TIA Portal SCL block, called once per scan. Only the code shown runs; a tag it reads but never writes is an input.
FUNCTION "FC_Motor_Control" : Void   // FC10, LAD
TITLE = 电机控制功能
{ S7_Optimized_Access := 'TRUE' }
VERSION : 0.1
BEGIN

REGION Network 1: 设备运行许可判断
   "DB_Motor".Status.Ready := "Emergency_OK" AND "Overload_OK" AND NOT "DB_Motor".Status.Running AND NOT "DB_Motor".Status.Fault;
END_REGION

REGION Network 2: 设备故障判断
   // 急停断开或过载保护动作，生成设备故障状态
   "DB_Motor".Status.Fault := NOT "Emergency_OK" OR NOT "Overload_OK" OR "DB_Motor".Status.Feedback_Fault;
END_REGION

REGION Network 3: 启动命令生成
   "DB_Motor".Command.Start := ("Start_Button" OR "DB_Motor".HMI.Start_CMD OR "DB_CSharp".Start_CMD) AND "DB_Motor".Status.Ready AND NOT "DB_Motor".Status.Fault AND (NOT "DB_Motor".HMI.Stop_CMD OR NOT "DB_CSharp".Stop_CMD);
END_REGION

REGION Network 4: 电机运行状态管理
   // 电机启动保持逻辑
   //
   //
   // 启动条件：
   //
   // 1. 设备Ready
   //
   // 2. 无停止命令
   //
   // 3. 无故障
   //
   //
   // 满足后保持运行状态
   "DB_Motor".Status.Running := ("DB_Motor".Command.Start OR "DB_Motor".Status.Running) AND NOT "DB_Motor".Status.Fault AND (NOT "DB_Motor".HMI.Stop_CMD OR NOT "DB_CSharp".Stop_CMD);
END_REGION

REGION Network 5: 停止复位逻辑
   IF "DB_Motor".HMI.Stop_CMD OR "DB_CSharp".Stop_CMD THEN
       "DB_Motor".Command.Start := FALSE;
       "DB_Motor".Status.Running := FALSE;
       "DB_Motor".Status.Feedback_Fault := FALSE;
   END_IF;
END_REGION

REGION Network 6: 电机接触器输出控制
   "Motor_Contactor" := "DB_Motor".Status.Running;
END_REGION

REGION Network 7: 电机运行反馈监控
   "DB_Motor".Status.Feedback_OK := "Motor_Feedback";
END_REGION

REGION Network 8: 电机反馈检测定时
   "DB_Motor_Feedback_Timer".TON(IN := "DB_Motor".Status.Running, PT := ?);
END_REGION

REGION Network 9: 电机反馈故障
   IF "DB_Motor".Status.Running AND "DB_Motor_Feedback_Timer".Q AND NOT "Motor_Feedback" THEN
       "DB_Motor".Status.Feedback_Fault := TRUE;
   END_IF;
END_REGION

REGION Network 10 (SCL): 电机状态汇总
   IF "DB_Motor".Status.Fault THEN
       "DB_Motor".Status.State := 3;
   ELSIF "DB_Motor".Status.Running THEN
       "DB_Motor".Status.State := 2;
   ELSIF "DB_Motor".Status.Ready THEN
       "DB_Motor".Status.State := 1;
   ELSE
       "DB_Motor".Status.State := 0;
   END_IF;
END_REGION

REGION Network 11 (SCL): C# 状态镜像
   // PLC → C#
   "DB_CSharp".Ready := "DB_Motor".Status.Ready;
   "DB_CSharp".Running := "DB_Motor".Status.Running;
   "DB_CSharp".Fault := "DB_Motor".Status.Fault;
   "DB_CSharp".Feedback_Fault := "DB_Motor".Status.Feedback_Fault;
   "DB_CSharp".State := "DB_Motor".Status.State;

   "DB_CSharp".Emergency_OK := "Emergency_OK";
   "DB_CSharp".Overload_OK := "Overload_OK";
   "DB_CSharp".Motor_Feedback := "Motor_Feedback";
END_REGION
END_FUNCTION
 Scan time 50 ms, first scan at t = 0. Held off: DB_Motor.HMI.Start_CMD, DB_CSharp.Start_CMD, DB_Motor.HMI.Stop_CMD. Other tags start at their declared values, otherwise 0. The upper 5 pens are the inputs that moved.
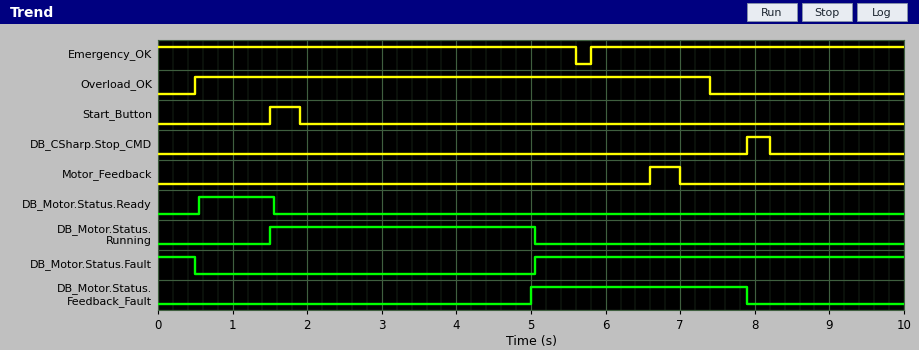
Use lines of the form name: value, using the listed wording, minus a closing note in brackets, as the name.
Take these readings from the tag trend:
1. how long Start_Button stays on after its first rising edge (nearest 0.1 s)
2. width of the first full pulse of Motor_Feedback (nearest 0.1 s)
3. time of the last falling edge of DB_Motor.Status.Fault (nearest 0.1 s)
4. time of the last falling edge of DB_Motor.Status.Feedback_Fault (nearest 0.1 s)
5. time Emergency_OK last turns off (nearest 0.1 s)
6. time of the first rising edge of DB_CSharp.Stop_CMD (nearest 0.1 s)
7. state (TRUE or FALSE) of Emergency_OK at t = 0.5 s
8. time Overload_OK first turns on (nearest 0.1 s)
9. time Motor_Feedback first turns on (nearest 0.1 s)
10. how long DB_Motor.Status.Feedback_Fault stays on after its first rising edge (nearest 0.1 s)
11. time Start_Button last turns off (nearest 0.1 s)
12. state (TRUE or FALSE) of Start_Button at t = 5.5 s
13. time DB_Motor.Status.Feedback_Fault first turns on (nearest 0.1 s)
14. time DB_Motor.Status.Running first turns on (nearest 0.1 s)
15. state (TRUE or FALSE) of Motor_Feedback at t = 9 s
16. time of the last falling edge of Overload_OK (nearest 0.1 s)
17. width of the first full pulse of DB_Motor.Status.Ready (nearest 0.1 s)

how long Start_Button stays on after its first rising edge: 0.4 s
width of the first full pulse of Motor_Feedback: 0.4 s
time of the last falling edge of DB_Motor.Status.Fault: 0.5 s
time of the last falling edge of DB_Motor.Status.Feedback_Fault: 7.9 s
time Emergency_OK last turns off: 5.6 s
time of the first rising edge of DB_CSharp.Stop_CMD: 7.9 s
state (TRUE or FALSE) of Emergency_OK at t = 0.5 s: TRUE
time Overload_OK first turns on: 0.5 s
time Motor_Feedback first turns on: 6.6 s
how long DB_Motor.Status.Feedback_Fault stays on after its first rising edge: 2.9 s
time Start_Button last turns off: 1.9 s
state (TRUE or FALSE) of Start_Button at t = 5.5 s: FALSE
time DB_Motor.Status.Feedback_Fault first turns on: 5.0 s
time DB_Motor.Status.Running first turns on: 1.5 s
state (TRUE or FALSE) of Motor_Feedback at t = 9 s: FALSE
time of the last falling edge of Overload_OK: 7.4 s
width of the first full pulse of DB_Motor.Status.Ready: 1.0 s
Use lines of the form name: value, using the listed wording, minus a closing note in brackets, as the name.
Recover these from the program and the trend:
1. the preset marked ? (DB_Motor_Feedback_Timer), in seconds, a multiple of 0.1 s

the preset marked ? (DB_Motor_Feedback_Timer), in seconds, a multiple of 0.1 s: 3.5 s
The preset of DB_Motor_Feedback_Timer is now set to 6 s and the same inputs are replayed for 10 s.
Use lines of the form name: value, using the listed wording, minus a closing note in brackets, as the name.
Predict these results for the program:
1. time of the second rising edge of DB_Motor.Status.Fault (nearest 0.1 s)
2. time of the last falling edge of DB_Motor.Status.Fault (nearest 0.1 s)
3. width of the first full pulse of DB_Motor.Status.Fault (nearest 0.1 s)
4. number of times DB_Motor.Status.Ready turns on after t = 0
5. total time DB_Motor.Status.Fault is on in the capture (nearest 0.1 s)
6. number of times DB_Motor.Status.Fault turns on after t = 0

time of the second rising edge of DB_Motor.Status.Fault: 7.4 s
time of the last falling edge of DB_Motor.Status.Fault: 5.8 s
width of the first full pulse of DB_Motor.Status.Fault: 0.2 s
number of times DB_Motor.Status.Ready turns on after t = 0: 2
total time DB_Motor.Status.Fault is on in the capture: 3.3 s
number of times DB_Motor.Status.Fault turns on after t = 0: 2
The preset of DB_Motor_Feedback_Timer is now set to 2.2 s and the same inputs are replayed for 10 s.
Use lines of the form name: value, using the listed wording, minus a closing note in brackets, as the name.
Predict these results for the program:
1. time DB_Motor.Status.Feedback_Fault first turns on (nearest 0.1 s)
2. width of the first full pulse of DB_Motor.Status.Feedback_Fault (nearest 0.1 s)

time DB_Motor.Status.Feedback_Fault first turns on: 3.7 s
width of the first full pulse of DB_Motor.Status.Feedback_Fault: 4.2 s
